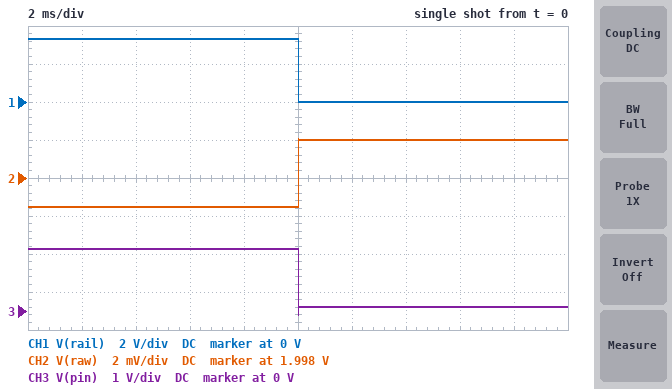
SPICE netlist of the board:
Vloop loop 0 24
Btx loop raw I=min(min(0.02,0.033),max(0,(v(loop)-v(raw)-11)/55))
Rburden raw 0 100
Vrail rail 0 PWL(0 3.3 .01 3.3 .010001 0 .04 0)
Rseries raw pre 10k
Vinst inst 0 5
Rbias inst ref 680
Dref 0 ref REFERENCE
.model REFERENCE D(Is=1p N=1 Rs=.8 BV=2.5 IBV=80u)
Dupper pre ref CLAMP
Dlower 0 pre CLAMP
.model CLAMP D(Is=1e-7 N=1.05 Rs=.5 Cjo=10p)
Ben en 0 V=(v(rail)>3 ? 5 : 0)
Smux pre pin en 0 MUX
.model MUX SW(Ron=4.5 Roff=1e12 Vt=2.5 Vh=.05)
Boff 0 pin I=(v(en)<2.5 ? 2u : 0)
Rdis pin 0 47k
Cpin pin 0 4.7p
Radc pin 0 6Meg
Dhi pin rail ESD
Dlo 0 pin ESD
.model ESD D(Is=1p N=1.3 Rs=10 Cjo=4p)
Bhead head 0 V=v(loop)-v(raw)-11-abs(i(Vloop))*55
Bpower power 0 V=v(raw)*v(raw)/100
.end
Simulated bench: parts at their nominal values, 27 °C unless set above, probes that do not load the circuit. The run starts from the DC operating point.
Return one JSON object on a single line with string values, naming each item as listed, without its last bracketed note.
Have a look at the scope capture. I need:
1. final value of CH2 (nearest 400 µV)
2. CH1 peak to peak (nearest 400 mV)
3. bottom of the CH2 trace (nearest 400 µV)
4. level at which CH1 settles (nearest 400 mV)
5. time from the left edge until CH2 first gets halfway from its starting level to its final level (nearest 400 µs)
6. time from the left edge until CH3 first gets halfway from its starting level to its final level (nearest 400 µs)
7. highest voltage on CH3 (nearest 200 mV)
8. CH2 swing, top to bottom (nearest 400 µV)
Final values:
{"final value of CH2": "2.0000 V", "CH1 peak to peak": "3.2 V", "bottom of the CH2 trace": "1.9964 V", "level at which CH1 settles": "0 V", "time from the left edge until CH2 first gets halfway from its starting level to its final level": "10.0 ms", "time from the left edge until CH3 first gets halfway from its starting level to its final level": "10.0 ms", "highest voltage on CH3": "1.6 V", "CH2 swing, top to bottom": "3.6 mV"}
